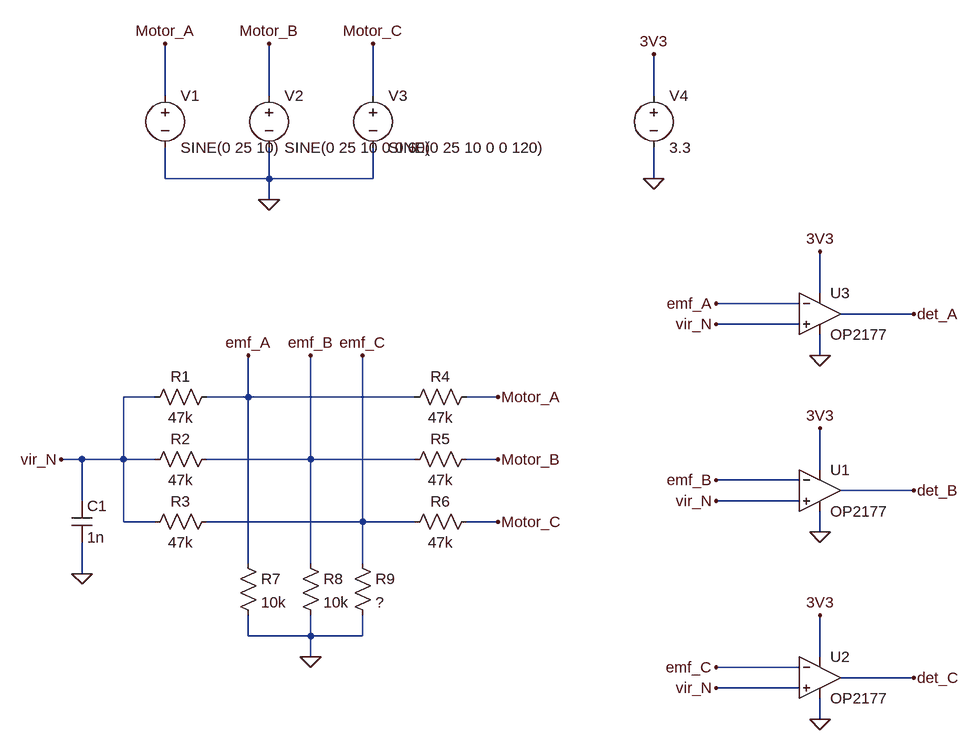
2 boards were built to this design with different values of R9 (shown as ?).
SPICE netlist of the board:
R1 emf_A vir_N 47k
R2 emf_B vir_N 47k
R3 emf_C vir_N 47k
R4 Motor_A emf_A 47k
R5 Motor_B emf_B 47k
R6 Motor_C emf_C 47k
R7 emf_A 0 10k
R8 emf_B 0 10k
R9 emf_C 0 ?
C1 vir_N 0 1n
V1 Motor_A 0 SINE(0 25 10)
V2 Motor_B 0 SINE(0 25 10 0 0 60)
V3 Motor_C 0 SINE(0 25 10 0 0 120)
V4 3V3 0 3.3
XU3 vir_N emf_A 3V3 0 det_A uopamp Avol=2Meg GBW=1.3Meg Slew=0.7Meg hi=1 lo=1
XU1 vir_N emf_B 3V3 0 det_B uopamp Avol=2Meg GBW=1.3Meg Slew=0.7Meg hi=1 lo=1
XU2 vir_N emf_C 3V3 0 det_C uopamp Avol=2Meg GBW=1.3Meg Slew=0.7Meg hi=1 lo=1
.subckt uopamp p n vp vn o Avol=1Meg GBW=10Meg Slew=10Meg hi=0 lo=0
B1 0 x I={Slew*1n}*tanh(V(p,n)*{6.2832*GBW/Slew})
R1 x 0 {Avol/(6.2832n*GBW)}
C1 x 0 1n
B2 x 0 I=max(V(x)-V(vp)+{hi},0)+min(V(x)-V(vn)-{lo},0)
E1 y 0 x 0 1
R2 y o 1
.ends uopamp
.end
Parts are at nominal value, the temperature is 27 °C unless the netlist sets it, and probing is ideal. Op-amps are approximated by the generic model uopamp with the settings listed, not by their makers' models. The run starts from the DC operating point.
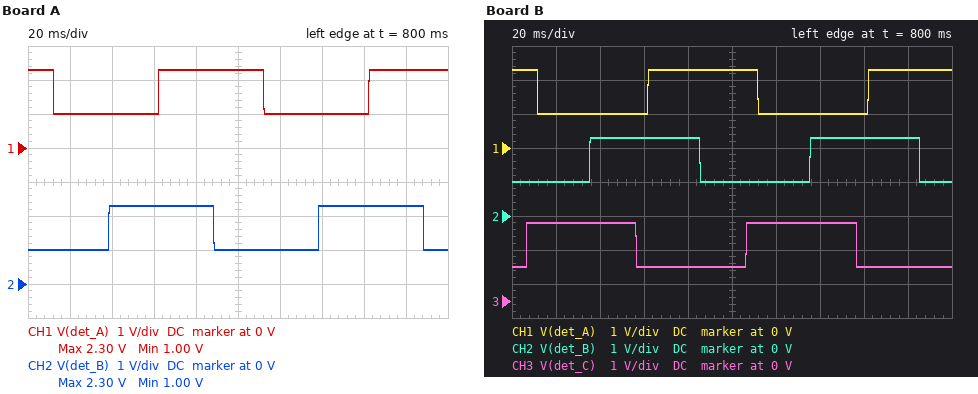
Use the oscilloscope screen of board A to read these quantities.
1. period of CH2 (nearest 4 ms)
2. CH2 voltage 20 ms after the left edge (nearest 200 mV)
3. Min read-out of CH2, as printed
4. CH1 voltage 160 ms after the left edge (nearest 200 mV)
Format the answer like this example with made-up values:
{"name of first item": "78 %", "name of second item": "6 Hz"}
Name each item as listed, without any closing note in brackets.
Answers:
{"period of CH2": "100 ms", "CH2 voltage 20 ms after the left edge": "1.0 V", "Min read-out of CH2, as printed": "1.00 V", "CH1 voltage 160 ms after the left edge": "1.0 V"}
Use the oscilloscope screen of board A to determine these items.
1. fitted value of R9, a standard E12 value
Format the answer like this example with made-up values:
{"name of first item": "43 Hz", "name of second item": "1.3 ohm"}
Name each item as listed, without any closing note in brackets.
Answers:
{"fitted value of R9, a standard E12 value": "15 kΩ"}
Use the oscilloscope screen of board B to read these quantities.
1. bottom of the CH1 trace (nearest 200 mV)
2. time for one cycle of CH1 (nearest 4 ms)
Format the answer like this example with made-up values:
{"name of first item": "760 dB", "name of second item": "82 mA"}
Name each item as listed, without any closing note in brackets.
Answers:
{"bottom of the CH1 trace": "1.0 V", "time for one cycle of CH1": "100 ms"}
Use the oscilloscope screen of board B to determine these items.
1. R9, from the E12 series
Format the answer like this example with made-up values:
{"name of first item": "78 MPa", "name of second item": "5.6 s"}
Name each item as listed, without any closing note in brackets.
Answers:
{"R9, from the E12 series": "12 kΩ"}
